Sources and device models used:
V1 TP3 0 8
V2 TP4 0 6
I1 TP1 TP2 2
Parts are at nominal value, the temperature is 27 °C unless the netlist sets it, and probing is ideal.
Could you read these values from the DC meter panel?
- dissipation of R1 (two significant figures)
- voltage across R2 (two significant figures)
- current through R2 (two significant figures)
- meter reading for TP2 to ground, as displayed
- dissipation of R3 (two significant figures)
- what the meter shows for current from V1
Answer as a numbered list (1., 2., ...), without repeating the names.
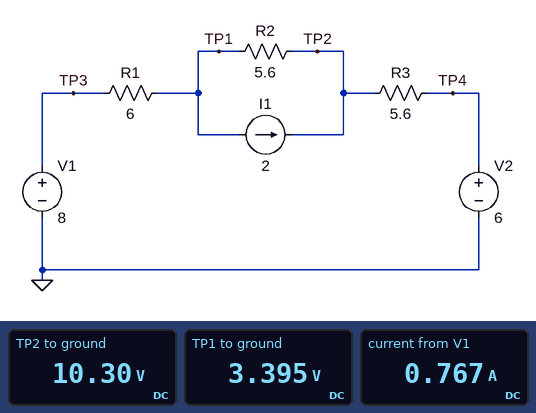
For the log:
1. 3.5 W
2. 6.9 V
3. 1.2 A
4. 10.30 V
5. 3.3 W
6. 0.767 A
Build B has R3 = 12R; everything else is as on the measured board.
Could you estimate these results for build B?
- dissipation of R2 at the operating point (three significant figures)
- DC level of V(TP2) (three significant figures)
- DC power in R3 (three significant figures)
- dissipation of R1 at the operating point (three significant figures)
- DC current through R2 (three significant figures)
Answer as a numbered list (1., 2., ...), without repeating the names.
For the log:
1. 11.6 W
2. 12.7 V
3. 3.75 W
4. 1.88 W
5. 1.44 A
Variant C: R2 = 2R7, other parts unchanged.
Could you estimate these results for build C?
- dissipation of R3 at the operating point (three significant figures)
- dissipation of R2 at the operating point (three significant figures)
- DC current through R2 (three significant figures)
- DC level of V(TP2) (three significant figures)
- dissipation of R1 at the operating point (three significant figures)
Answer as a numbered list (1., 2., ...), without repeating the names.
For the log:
1. 1.50 W
2. 5.93 W
3. 1.48 A
4. 8.90 V
5. 1.61 W
